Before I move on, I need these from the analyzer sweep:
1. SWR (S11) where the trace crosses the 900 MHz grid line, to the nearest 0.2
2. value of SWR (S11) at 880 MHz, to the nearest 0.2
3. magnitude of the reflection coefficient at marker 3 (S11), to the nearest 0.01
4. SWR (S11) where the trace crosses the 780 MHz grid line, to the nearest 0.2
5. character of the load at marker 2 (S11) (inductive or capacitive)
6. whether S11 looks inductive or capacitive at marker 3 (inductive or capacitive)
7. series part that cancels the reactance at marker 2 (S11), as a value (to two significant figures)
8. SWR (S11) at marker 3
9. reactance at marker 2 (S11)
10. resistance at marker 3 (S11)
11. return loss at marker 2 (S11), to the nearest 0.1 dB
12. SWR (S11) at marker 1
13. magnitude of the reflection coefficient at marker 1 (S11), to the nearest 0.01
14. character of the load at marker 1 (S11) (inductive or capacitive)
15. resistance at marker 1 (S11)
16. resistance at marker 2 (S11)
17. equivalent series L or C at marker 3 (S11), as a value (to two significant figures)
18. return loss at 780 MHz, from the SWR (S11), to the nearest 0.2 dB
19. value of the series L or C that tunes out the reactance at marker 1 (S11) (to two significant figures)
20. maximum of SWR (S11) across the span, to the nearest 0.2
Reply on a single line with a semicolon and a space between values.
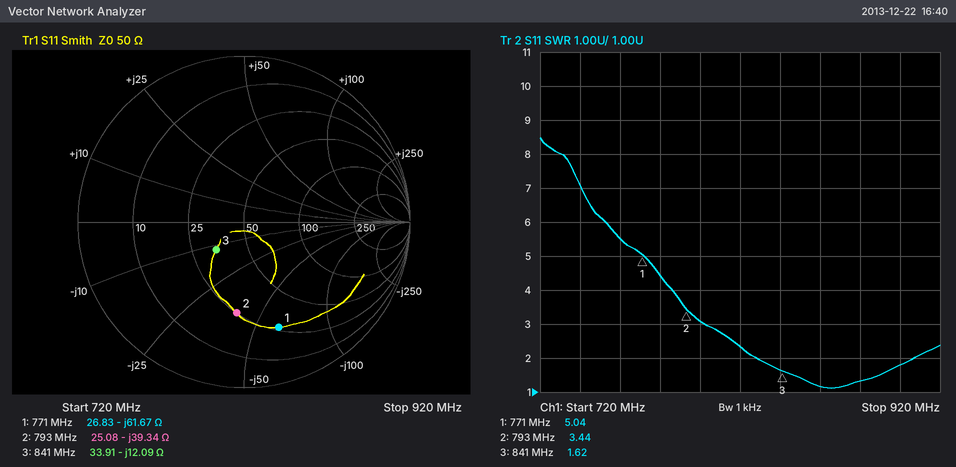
1.8; 1.4; 0.24; 4.4; capacitive; capacitive; 7.9 nH; 1.62; -39.34 Ω; 33.91 Ω; 5.2 dB; 5.04; 0.67; capacitive; 26.83 Ω; 25.08 Ω; 16 pF; 4.0 dB; 13 nH; 8.4
